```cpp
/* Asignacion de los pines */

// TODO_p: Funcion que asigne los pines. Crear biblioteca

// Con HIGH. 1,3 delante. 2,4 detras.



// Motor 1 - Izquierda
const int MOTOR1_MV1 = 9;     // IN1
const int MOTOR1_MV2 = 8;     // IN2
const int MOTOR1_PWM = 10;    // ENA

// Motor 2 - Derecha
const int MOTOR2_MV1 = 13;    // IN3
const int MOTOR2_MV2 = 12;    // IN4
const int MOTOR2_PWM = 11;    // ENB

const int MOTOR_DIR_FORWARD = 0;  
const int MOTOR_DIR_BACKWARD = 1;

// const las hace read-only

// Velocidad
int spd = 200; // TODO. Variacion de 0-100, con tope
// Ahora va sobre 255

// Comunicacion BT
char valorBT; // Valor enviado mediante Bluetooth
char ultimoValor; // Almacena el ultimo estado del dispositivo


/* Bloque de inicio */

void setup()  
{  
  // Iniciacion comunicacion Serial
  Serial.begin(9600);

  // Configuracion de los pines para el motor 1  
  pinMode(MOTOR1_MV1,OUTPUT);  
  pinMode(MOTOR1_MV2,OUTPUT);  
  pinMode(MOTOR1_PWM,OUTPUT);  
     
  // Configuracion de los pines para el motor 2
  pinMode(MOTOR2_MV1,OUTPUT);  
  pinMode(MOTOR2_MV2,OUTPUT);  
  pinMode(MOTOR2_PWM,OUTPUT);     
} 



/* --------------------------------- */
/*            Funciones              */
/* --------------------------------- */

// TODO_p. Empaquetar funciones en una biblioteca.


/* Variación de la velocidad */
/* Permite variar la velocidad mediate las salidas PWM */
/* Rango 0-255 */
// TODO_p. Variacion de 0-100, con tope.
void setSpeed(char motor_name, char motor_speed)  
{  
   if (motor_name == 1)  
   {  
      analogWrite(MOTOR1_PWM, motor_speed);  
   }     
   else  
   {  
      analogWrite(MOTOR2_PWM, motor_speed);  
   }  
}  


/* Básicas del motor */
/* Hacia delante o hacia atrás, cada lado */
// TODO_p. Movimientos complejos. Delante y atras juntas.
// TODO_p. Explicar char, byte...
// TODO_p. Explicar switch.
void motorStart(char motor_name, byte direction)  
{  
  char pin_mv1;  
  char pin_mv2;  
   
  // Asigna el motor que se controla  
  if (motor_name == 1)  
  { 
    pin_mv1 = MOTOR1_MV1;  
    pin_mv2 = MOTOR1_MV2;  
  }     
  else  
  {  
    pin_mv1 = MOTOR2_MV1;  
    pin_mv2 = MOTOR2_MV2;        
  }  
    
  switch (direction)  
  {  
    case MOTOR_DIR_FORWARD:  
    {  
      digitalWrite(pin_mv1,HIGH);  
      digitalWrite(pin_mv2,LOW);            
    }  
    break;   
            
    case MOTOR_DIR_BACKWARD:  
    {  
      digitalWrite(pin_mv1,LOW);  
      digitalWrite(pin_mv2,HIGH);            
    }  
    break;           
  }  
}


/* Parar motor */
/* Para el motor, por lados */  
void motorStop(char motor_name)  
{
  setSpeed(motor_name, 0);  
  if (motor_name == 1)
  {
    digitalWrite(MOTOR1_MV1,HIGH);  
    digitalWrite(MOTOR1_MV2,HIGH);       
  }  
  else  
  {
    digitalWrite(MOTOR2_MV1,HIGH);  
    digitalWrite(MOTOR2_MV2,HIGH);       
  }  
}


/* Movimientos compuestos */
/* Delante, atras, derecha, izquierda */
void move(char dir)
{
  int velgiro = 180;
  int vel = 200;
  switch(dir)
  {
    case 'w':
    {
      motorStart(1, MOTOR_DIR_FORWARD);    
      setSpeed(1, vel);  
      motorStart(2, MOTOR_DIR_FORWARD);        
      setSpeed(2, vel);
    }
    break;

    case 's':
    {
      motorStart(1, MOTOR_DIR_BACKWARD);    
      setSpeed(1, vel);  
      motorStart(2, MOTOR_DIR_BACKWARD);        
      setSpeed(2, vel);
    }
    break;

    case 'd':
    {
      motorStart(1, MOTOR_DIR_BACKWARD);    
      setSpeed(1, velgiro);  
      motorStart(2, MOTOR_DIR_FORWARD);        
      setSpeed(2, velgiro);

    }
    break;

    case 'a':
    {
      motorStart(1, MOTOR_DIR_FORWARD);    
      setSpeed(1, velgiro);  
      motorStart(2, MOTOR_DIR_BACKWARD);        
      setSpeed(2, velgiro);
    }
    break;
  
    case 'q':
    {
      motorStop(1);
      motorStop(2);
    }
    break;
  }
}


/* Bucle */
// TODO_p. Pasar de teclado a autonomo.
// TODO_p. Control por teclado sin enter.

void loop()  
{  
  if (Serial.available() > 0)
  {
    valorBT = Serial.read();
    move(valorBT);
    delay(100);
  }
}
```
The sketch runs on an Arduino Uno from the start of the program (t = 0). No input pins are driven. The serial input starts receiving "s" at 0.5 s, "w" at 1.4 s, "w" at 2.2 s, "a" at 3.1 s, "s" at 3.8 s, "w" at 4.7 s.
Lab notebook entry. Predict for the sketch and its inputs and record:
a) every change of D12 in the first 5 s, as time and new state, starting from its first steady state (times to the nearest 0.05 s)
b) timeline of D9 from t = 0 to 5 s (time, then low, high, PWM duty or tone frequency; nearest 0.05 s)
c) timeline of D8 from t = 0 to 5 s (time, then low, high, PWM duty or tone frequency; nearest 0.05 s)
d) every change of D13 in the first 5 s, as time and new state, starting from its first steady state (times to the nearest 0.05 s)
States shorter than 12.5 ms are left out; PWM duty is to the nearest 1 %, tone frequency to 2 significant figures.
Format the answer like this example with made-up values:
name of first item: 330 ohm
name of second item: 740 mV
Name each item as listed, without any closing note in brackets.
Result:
every change of D12 in the first 5 s, as time and new state, starting from its first steady state: 0 s low; 0.5 s high; 1.4 s low; 3.1 s high; 4.7 s low
timeline of D9 from t = 0 to 5 s: 0 s low; 1.4 s high; 3.8 s low; 4.7 s high
timeline of D8 from t = 0 to 5 s: 0 s low; 0.5 s high; 1.4 s low; 3.8 s high; 4.7 s low
every change of D13 in the first 5 s, as time and new state, starting from its first steady state: 0 s low; 1.4 s high; 3.1 s low; 4.7 s high
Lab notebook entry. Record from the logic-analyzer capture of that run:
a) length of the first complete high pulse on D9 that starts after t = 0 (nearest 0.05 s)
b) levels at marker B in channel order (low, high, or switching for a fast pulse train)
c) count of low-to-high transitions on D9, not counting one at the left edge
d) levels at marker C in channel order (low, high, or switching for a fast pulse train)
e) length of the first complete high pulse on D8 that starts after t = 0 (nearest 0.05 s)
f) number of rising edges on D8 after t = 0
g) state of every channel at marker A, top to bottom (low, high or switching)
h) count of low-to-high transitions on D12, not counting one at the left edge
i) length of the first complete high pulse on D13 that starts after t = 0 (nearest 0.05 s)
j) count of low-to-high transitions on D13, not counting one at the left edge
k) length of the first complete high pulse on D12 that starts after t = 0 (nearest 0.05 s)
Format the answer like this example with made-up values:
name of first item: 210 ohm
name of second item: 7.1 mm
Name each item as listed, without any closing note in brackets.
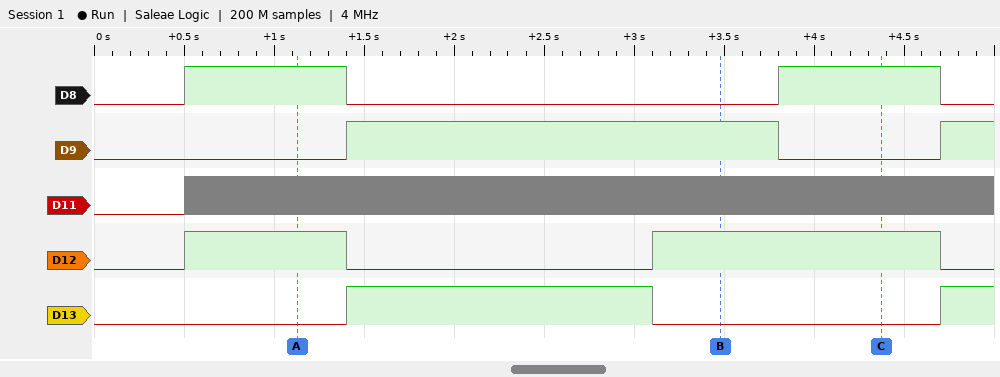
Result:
length of the first complete high pulse on D9 that starts after t = 0: 2.40 s
levels at marker B in channel order: D8 low, D9 high, D11 switching, D12 high, D13 low
count of low-to-high transitions on D9, not counting one at the left edge: 2
levels at marker C in channel order: D8 high, D9 low, D11 switching, D12 high, D13 low
length of the first complete high pulse on D8 that starts after t = 0: 0.90 s
number of rising edges on D8 after t = 0: 2
state of every channel at marker A, top to bottom: D8 high, D9 low, D11 switching, D12 high, D13 low
count of low-to-high transitions on D12, not counting one at the left edge: 2
length of the first complete high pulse on D13 that starts after t = 0: 1.70 s
count of low-to-high transitions on D13, not counting one at the left edge: 2
length of the first complete high pulse on D12 that starts after t = 0: 0.90 s
